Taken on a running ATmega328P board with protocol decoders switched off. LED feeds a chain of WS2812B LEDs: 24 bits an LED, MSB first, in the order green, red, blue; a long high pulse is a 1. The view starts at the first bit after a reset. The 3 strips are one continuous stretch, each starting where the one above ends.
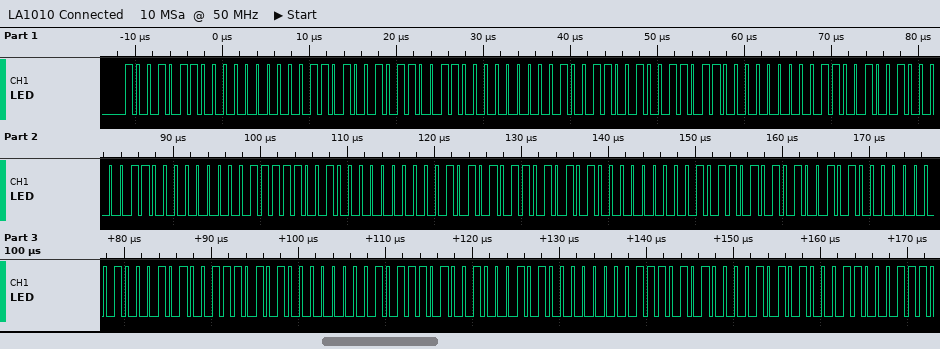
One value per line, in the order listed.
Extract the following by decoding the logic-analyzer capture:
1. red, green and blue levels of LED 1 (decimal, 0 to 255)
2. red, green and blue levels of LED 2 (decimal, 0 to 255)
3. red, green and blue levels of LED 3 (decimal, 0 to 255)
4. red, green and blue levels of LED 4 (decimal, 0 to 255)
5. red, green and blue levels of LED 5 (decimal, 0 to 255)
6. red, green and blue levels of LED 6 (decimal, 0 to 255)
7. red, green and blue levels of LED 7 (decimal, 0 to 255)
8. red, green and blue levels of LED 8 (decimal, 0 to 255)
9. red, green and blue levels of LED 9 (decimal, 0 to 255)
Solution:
0, 150, 105
0, 102, 153
0, 54, 201
0, 6, 249
42, 0, 213
90, 0, 165
138, 0, 117
186, 0, 69
234, 0, 21
